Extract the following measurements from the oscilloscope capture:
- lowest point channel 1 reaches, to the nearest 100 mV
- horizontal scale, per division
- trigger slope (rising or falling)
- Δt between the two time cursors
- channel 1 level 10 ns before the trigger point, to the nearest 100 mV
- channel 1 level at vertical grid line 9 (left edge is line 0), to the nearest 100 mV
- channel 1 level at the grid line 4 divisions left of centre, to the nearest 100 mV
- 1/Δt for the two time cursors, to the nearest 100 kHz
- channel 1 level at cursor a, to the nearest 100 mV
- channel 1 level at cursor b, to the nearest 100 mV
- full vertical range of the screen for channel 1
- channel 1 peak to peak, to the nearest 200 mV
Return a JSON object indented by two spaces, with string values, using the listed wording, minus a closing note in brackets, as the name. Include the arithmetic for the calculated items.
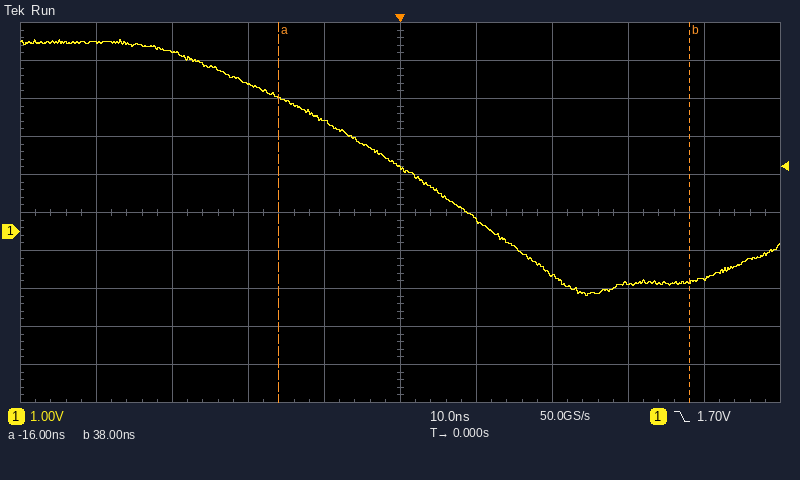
{
  "lowest point channel 1 reaches, to the nearest 100 mV": "-1.7 V",
  "horizontal scale, per division": "10 ns",
  "trigger slope": "falling",
  "Δt between the two time cursors": "38 ns − (-16 ns) = 54 ns",
  "channel 1 level 10 ns before the trigger point, to the nearest 100 mV": "2.9 V",
  "channel 1 level at vertical grid line 9 (left edge is line 0), to the nearest 100 mV": "-1.2 V",
  "channel 1 level at the grid line 4 divisions left of centre, to the nearest 100 mV": "5.0 V",
  "1/Δt for the two time cursors, to the nearest 100 kHz": "1 / 54 ns ≈ 18.5 MHz",
  "channel 1 level at cursor a, to the nearest 100 mV": "3.5 V",
  "channel 1 level at cursor b, to the nearest 100 mV": "-1.3 V",
  "full vertical range of the screen for channel 1": "10 V",
  "channel 1 peak to peak, to the nearest 200 mV": "6.8 V"
}
